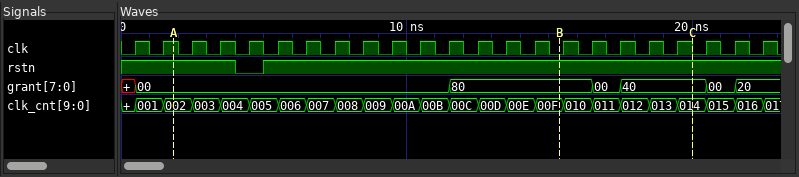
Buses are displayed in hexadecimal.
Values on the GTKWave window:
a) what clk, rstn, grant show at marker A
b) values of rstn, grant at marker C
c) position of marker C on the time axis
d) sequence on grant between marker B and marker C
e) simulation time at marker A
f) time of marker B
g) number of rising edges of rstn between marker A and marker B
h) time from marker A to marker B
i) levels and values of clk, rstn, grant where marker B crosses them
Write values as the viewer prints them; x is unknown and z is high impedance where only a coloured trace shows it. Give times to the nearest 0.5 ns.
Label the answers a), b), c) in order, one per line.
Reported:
a) clk=1, rstn=1, grant=00
b) rstn=1, grant=40
c) 20 ns
d) 80, 00, 40
e) 2 ns
f) 15.5 ns
g) 1
h) 13.5 ns
i) clk=0, rstn=1, grant=80
